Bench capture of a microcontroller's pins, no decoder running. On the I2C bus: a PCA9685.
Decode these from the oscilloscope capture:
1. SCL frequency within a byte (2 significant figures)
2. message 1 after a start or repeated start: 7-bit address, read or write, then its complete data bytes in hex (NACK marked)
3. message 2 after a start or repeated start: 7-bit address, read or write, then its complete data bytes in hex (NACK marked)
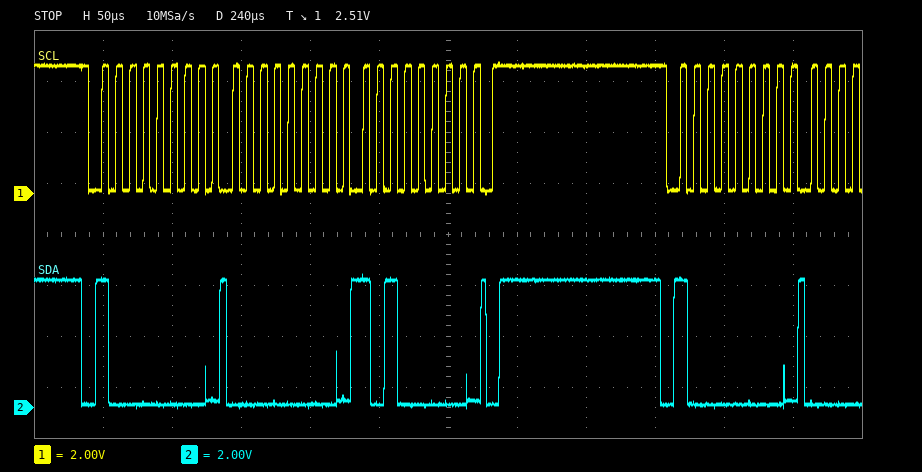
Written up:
100 kHz
0x40 write: 00 A0
0x40 write
